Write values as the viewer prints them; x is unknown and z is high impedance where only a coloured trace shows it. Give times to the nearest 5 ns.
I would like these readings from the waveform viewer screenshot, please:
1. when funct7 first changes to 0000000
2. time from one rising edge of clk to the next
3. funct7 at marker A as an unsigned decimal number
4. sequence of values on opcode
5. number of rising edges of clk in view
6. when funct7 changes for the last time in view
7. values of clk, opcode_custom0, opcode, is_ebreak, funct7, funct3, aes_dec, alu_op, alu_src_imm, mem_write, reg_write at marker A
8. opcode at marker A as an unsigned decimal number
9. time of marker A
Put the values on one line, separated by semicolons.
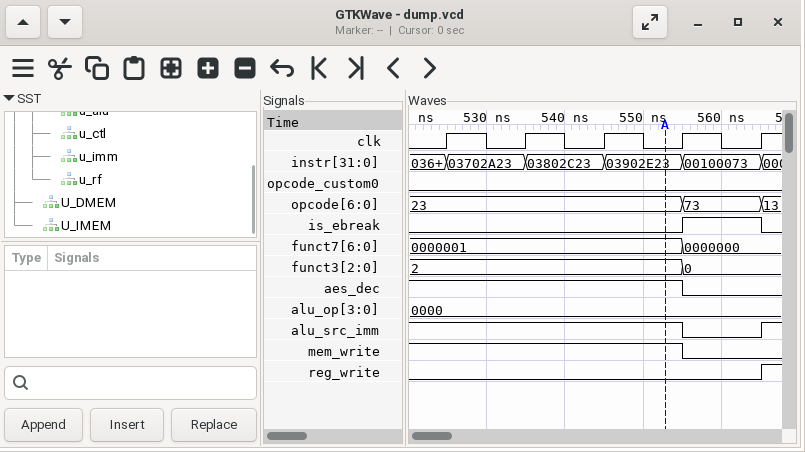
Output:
555 ns; 10 ns; 1; 23, 73, 13; 5; 555 ns; clk=0, opcode_custom0=0, opcode=23, is_ebreak=0, funct7=0000001, funct3=2, aes_dec=1, alu_op=0000, alu_src_imm=1, mem_write=1, reg_write=0; 35; 555 ns
